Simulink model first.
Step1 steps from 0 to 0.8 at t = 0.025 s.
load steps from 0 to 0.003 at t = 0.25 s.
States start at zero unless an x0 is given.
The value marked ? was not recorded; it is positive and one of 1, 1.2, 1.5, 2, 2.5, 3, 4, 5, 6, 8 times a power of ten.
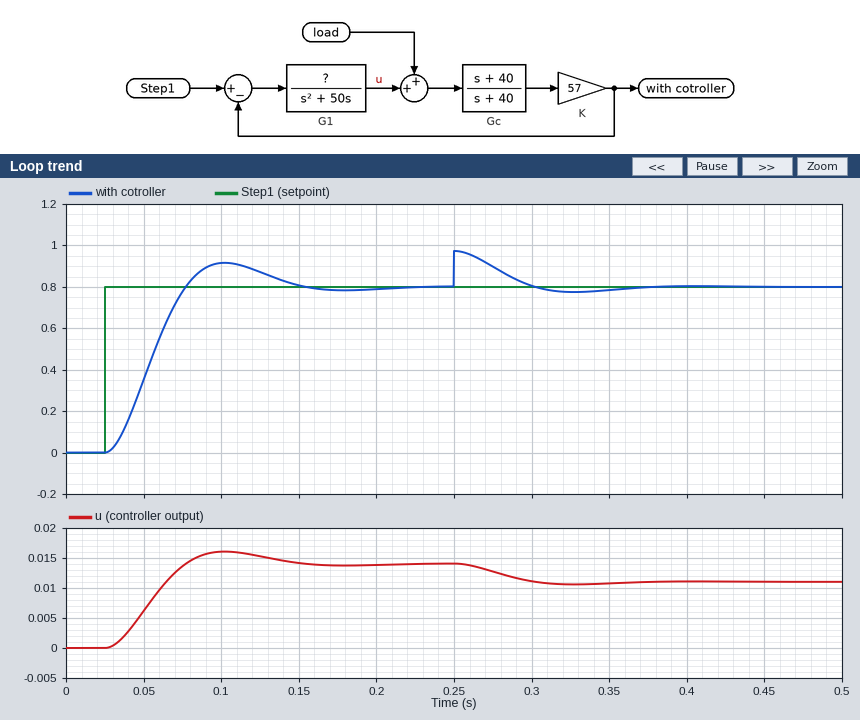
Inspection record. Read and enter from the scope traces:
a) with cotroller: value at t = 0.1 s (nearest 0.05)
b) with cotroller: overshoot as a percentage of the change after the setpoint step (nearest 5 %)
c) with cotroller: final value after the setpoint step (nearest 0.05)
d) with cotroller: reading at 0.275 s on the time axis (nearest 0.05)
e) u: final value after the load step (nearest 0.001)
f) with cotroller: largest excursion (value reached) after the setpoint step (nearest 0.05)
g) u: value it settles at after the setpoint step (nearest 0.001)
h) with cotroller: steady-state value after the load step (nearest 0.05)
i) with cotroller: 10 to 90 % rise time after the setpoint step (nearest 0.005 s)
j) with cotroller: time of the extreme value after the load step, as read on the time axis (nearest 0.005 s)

0.90
15 %
0.80
0.90
0.011
0.90
0.014
0.80
0.035 s
0.250 s
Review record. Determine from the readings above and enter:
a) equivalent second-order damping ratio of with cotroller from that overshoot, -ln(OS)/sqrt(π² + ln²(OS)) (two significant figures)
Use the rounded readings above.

0.52
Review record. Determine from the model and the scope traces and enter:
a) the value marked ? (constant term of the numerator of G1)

40
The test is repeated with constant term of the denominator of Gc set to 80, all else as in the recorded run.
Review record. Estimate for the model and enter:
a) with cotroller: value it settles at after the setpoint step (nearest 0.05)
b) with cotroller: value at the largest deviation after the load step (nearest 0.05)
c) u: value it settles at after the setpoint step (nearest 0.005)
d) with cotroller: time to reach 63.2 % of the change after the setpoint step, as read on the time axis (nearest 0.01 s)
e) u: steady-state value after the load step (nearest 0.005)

0.80
0.95
0.030
0.07 s
0.025
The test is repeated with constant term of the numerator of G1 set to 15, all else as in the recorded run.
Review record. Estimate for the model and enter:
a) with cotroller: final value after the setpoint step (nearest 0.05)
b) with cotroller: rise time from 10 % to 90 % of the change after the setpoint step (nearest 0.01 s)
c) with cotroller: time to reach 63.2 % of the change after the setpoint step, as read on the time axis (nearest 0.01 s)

0.80
0.09 s
0.09 s
